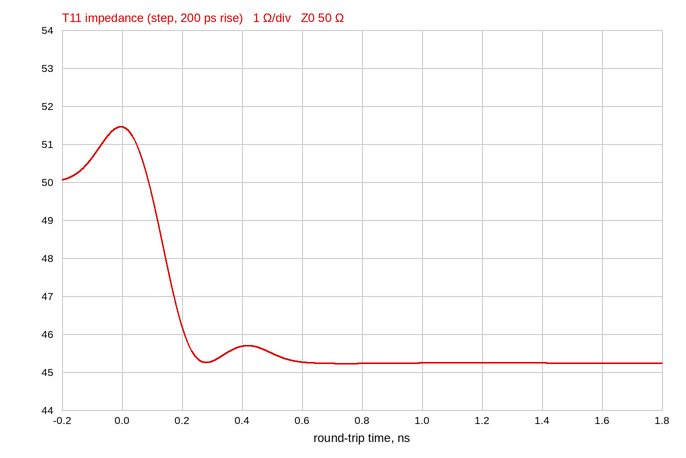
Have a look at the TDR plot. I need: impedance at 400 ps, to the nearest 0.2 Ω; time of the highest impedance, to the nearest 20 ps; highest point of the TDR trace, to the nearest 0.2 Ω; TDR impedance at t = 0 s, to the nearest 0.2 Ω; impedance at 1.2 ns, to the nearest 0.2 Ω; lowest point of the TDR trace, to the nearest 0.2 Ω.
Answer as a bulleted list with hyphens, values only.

- 45.6 Ω
- 0 ps
- 51.4 Ω
- 51.4 Ω
- 45.2 Ω
- 45.2 Ω
